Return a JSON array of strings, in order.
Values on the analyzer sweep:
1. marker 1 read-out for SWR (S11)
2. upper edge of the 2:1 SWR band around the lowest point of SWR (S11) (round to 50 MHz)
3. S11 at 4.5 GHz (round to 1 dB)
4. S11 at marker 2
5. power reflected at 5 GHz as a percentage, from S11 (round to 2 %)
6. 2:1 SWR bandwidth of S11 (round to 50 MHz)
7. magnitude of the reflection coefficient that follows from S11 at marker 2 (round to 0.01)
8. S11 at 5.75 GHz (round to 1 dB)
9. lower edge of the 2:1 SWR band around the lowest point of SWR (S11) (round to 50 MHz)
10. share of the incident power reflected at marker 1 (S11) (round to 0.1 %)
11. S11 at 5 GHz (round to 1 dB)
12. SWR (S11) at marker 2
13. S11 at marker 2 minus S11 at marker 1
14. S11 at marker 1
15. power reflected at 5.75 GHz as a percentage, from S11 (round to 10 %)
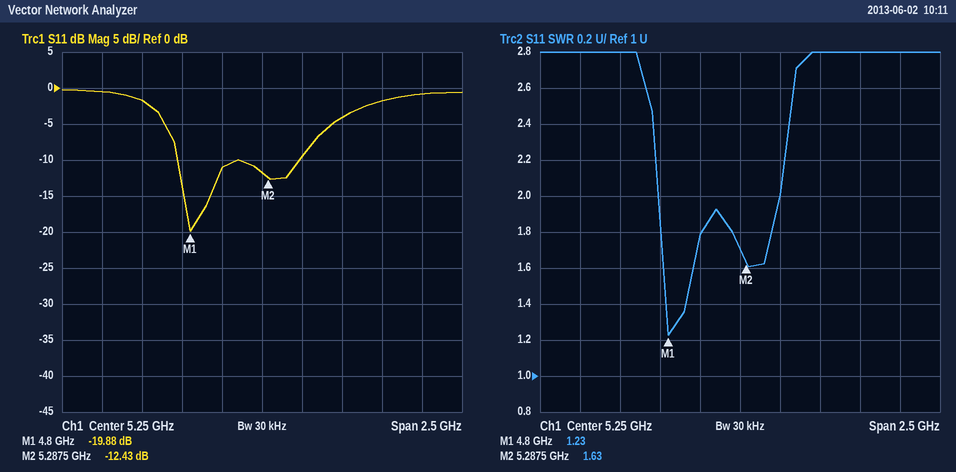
["1.23", "5.50 GHz", "-2 dB", "-12.43 dB", "8 %", "750 MHz", "0.24", "-4 dB", "4.75 GHz", "1.0 %", "-11 dB", "1.63", "7.45 dB", "-19.88 dB", "40 %"]
